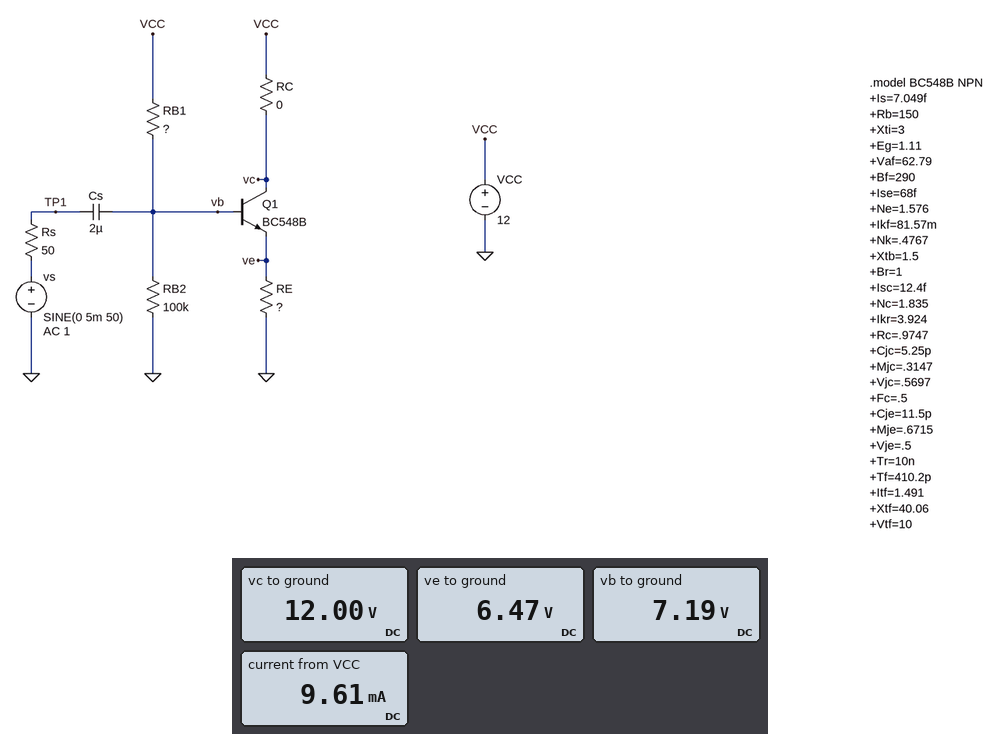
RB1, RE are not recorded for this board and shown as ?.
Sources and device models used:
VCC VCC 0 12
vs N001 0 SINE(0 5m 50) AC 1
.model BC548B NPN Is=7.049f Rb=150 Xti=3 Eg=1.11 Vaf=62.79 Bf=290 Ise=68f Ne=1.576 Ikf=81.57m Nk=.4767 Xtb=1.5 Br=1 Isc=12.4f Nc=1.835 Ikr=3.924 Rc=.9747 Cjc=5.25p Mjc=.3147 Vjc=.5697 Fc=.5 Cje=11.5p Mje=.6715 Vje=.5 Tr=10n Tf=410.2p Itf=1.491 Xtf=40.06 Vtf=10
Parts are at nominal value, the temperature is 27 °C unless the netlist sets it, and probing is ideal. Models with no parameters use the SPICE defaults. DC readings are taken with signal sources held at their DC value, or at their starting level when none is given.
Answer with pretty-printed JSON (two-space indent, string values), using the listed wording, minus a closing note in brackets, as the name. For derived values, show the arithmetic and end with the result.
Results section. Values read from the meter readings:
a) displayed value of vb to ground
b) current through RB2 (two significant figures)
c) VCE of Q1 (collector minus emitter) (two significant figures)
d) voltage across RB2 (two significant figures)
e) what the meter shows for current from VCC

{
  "displayed value of vb to ground": "7.19 V",
  "current through RB2": "(7.19 V) / 100 kΩ = 72 µA",
  "VCE of Q1 (collector minus emitter)": "12 V - 6.47 V = 5.5 V",
  "voltage across RB2": "7.19 V = 7.2 V",
  "what the meter shows for current from VCC": "9.61 mA"
}
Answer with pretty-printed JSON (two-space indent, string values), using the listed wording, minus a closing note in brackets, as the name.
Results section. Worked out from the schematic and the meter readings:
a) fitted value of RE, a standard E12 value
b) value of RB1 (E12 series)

{
  "fitted value of RE, a standard E12 value": "820 Ω",
  "value of RB1": "47 kΩ"
}
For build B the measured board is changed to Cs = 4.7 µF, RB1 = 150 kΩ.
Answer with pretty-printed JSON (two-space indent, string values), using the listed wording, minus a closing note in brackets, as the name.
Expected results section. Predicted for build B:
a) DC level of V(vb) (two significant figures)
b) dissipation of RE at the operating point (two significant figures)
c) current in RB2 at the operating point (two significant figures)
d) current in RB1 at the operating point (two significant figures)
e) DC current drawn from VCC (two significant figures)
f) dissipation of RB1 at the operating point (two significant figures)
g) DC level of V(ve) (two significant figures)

{
  "DC level of V(vb)": "3.9 V",
  "dissipation of RE at the operating point": "13 mW",
  "current in RB2 at the operating point": "39 µA",
  "current in RB1 at the operating point": "54 µA",
  "DC current drawn from VCC": "3.9 mA",
  "dissipation of RB1 at the operating point": "430 µW",
  "DC level of V(ve)": "3.2 V"
}
